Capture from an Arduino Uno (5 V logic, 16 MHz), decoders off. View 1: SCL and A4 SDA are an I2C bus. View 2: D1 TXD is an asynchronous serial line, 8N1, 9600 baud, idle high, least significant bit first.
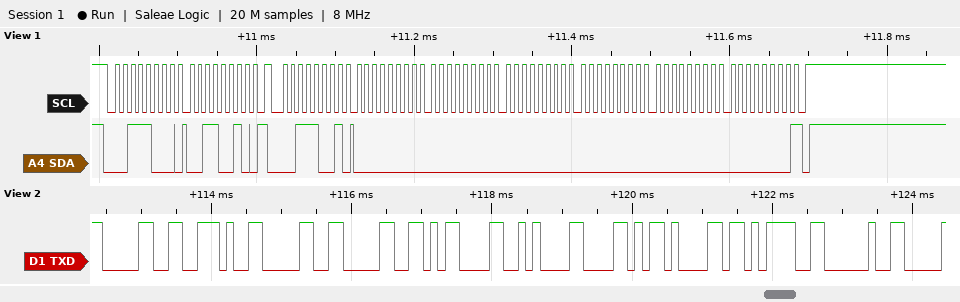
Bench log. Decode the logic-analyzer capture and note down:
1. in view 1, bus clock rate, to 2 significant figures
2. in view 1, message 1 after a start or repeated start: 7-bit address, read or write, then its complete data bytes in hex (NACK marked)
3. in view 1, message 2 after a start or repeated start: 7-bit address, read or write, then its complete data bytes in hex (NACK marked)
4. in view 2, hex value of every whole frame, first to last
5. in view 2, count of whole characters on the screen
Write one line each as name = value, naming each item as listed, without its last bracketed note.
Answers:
in view 1, bus clock rate, to 2 significant figures = 100 kHz
in view 1, message 1 after a start or repeated start: 7-bit address, read or write, then its complete data bytes in hex = 0x1C write: 32
in view 1, message 2 after a start or repeated start: 7-bit address, read or write, then its complete data bytes in hex = 0x1C read: 00 00 00 00 00 00 NACK
in view 2, hex value of every whole frame, first to last = 30 2E 30 30 0D 0A 58 61 3D 20
in view 2, count of whole characters on the screen = 10
